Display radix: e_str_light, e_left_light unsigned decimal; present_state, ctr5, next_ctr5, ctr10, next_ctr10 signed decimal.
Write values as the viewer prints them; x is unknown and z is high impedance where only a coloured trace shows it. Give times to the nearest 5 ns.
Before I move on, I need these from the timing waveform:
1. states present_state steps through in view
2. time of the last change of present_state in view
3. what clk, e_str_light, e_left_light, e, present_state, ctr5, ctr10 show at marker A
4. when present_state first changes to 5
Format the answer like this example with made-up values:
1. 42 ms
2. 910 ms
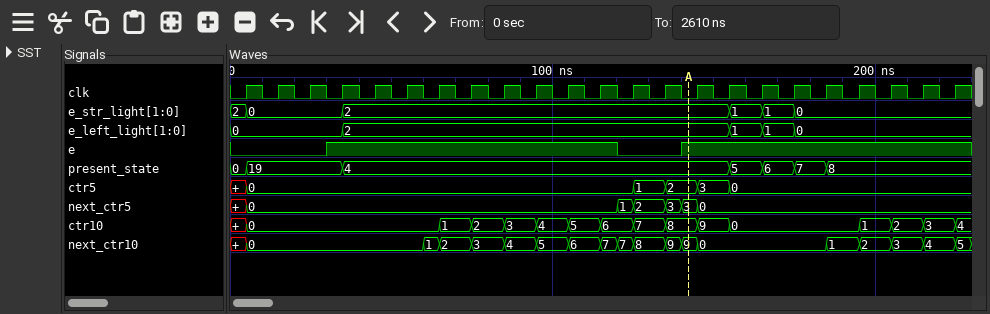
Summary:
1. 0, 19, 4, 5, 6, 7, 8
2. 185 ns
3. clk=0, e_str_light=2, e_left_light=2, e=1, present_state=4, ctr5=2, ctr10=8
4. 155 ns
